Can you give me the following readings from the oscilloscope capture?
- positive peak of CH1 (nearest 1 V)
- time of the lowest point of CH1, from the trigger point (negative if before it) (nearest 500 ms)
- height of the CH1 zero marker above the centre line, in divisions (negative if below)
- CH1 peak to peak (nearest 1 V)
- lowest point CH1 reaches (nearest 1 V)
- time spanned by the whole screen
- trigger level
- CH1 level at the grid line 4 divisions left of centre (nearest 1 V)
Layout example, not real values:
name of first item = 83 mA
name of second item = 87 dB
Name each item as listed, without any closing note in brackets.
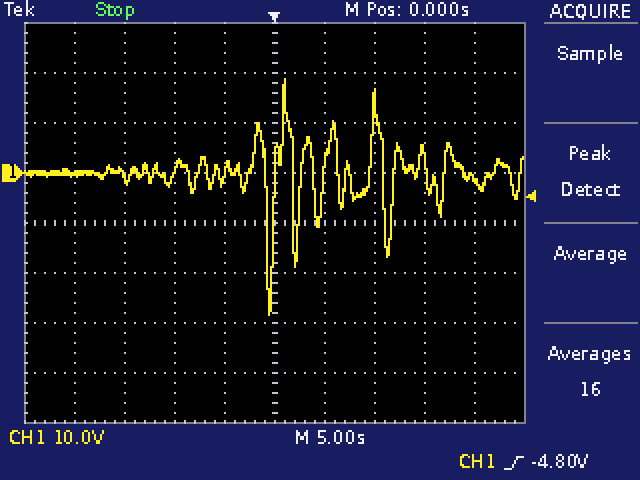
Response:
positive peak of CH1 = 19 V
time of the lowest point of CH1, from the trigger point (negative if before it) = -500 ms
height of the CH1 zero marker above the centre line, in divisions = +1.0 div
CH1 peak to peak = 47 V
lowest point CH1 reaches = -28 V
time spanned by the whole screen = 50 s
trigger level = -4.80 V
CH1 level at the grid line 4 divisions left of centre = 0 V
